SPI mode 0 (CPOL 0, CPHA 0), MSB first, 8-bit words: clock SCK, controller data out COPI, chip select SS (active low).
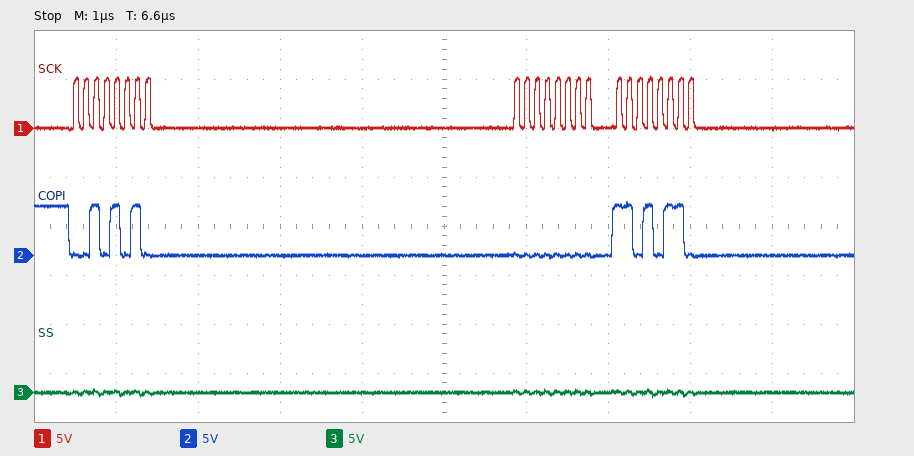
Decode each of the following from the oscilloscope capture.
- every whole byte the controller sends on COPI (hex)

2A 00 D6
